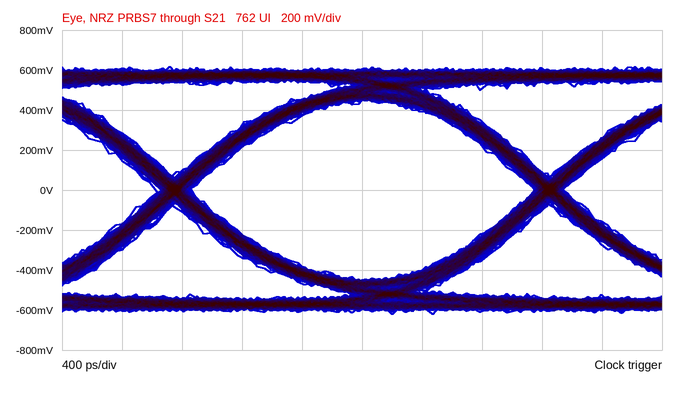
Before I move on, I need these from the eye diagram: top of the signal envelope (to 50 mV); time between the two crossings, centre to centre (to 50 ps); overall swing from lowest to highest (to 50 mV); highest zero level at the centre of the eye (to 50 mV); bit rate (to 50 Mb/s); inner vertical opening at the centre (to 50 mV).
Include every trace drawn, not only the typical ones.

600 mV
2.50 ns
1.25 V
-450 mV
400 Mb/s
900 mV
